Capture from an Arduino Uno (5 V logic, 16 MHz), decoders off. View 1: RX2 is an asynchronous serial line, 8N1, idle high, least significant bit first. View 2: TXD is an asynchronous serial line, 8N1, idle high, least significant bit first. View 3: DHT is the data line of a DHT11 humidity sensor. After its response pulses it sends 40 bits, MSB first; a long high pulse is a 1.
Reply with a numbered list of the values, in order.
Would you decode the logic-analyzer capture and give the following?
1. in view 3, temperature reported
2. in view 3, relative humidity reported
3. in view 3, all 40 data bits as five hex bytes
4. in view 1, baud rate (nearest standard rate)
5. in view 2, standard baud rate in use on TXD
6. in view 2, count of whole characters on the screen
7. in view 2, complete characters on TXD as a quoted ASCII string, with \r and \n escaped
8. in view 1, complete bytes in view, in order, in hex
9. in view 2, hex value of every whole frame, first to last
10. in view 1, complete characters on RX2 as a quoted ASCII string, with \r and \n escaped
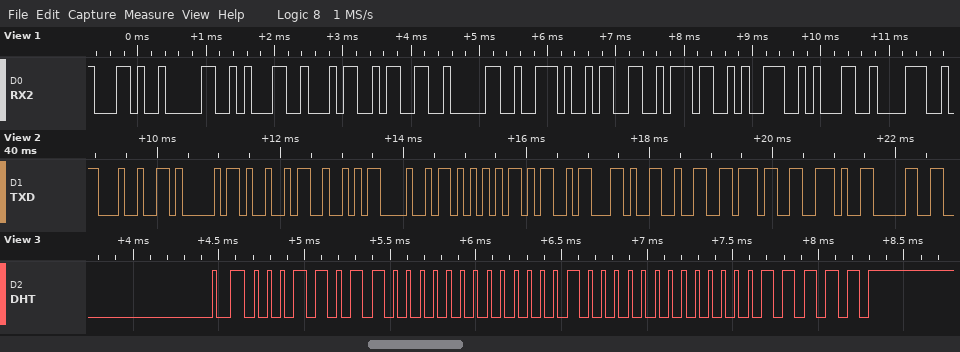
1. 4.0 °C
2. 27 %
3. 1B 00 04 00 1F
4. 9600 baud
5. 9600 baud
6. 12
7. "$AIRHUM,27.0"
8. 2C 30 31 34 33 30 2E 33 37 39 31 38
9. 24 41 49 52 48 55 4D 2C 32 37 2E 30
10. ",01430.37918"
